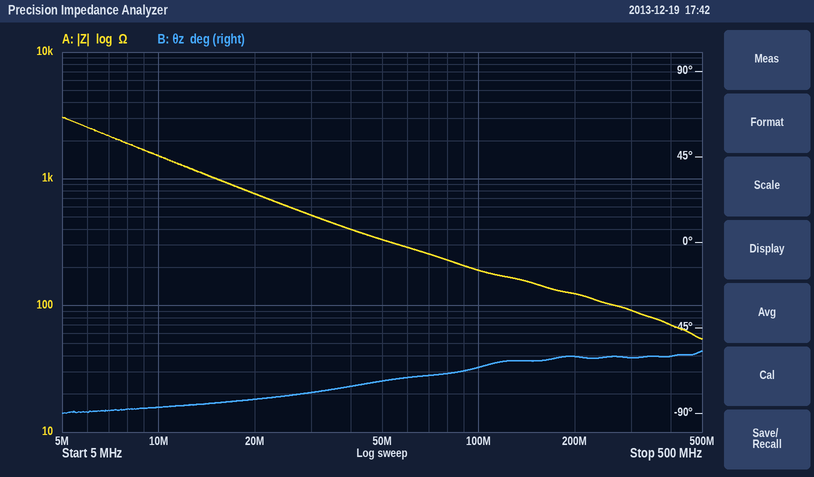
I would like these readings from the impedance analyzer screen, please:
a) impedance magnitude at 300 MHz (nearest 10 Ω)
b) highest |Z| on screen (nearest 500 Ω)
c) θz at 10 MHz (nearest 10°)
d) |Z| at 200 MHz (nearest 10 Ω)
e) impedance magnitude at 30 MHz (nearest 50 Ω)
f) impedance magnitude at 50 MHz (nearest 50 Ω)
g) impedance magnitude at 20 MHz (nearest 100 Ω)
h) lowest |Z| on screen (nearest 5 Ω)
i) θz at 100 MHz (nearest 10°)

90 Ω
3.0 kΩ
-90°
120 Ω
500 Ω
350 Ω
800 Ω
55 Ω
-70°
